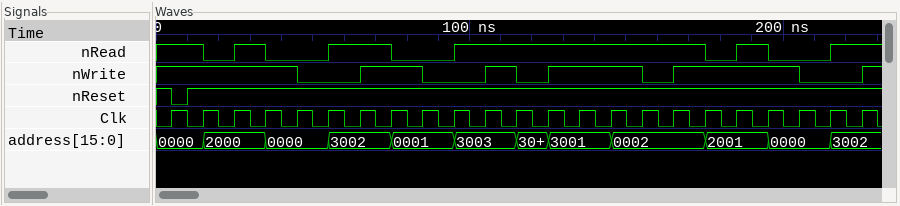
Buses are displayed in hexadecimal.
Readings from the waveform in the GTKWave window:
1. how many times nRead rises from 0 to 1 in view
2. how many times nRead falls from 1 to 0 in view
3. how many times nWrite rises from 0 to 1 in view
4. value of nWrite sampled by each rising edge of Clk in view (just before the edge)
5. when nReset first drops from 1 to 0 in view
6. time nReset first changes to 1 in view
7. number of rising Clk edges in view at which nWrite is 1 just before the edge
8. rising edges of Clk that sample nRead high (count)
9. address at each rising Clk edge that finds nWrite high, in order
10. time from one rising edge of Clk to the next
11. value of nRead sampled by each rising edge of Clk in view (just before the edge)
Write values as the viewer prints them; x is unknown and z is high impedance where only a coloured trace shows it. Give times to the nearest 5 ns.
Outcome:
5
5
5
1 1 1 1 1 0 0 1 1 0 0 1 0 1 1 1 0 1 1 1 1 0 0
5 ns
10 ns
15
15
0000, 0000, 2000, 2000, 0000, 3002, 0001, 3003, 3001, 3001, 0002, 0002, 2001, 2001, 0000
10 ns
1 1 0 1 0 0 1 1 0 0 1 1 1 1 1 1 1 1 0 1 0 0 1
